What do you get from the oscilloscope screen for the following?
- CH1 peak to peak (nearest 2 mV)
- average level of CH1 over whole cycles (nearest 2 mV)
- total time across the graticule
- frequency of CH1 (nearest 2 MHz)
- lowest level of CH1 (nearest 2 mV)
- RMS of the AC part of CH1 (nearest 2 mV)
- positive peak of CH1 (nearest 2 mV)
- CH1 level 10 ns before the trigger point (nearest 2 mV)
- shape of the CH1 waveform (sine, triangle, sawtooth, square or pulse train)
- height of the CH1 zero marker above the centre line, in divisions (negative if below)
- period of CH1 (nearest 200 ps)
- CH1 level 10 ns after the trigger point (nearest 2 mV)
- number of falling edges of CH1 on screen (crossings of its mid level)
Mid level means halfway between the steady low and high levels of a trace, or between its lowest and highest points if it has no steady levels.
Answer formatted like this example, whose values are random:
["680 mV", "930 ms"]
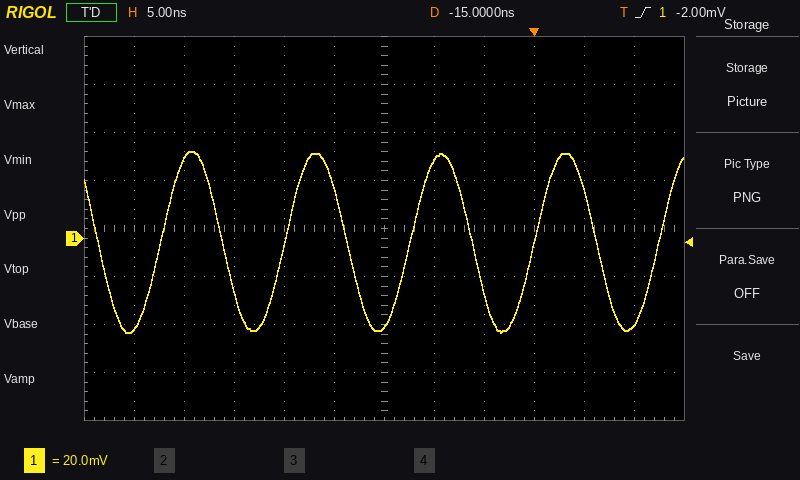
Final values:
["76 mV", "-2 mV", "60 ns", "80 MHz", "-40 mV", "26 mV", "36 mV", "32 mV", "sine", "-0.2 div", "12.4 ns", "-36 mV", "5"]
